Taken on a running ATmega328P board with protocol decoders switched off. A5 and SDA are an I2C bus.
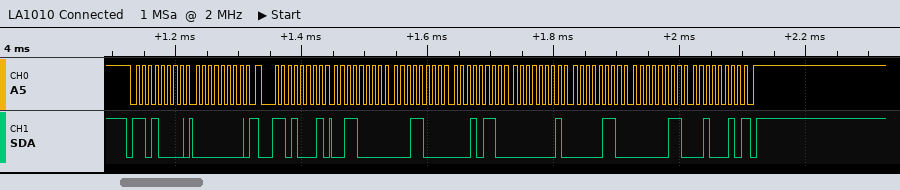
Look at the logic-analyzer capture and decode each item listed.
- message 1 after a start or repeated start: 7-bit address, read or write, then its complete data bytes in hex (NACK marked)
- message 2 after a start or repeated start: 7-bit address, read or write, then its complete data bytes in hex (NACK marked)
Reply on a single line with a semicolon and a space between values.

0x68 write: 00; 0x68 read: 30 18 16 01 06 03 22 NACK
